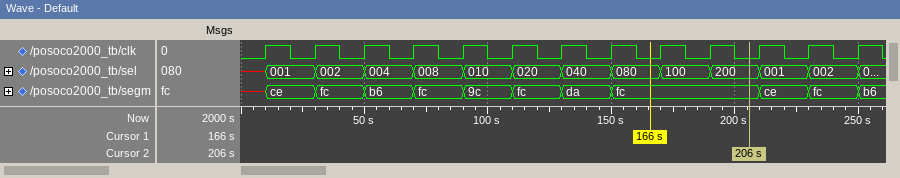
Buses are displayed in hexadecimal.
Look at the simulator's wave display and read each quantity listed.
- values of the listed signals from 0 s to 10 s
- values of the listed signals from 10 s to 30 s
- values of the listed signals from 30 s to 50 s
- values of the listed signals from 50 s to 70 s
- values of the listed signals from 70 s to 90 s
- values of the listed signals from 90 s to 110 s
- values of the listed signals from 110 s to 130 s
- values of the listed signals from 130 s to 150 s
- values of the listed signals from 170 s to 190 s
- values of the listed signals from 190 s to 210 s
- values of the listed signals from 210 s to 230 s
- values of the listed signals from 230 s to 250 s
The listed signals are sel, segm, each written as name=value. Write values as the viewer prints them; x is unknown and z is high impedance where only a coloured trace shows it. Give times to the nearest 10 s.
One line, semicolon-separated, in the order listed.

sel=x, segm=x; sel=001, segm=ce; sel=002, segm=fc; sel=004, segm=b6; sel=008, segm=fc; sel=010, segm=9c; sel=020, segm=fc; sel=040, segm=da; sel=100, segm=fc; sel=200, segm=fc; sel=001, segm=ce; sel=002, segm=fc
